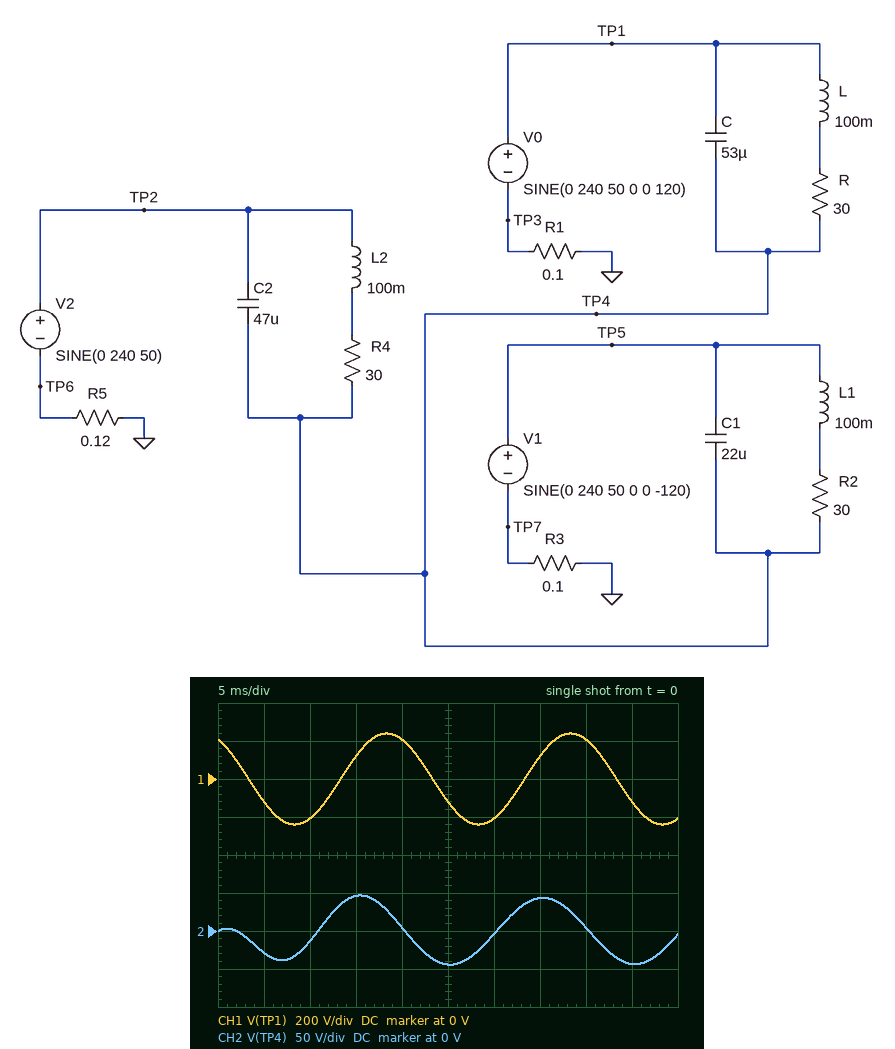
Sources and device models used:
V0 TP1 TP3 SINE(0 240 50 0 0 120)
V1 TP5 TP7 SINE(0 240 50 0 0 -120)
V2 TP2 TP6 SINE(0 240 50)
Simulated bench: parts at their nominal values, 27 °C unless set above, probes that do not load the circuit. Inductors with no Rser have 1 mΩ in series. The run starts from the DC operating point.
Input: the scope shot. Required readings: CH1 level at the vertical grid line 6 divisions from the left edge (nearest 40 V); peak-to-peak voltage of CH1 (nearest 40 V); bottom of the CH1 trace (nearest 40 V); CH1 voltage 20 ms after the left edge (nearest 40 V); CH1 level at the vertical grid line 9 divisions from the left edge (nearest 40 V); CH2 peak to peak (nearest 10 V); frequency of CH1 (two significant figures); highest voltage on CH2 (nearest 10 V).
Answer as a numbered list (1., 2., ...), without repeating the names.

1. -200 V
2. 480 V
3. -240 V
4. 200 V
5. -120 V
6. 90 V
7. 50 Hz
8. 50 V
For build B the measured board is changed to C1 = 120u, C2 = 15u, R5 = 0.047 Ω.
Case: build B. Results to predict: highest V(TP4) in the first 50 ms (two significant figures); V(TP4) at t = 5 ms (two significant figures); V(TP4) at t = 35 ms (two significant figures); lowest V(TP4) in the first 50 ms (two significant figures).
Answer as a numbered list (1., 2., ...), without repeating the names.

1. 140 V
2. 13 V
3. -67 V
4. -140 V
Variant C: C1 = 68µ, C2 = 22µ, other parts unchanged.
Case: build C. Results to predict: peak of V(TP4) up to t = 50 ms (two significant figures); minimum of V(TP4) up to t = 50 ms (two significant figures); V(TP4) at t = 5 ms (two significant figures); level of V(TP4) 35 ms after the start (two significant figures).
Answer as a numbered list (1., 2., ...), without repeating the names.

1. 65 V
2. -67 V
3. -6.8 V
4. -27 V
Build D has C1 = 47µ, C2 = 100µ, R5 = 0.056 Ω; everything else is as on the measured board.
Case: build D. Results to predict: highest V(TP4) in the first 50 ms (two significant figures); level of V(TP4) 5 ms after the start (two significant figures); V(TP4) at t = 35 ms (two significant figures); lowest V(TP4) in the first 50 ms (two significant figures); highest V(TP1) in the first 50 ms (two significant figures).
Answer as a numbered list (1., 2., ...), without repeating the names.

1. 77 V
2. 25 V
3. -13 V
4. -77 V
5. 240 V
